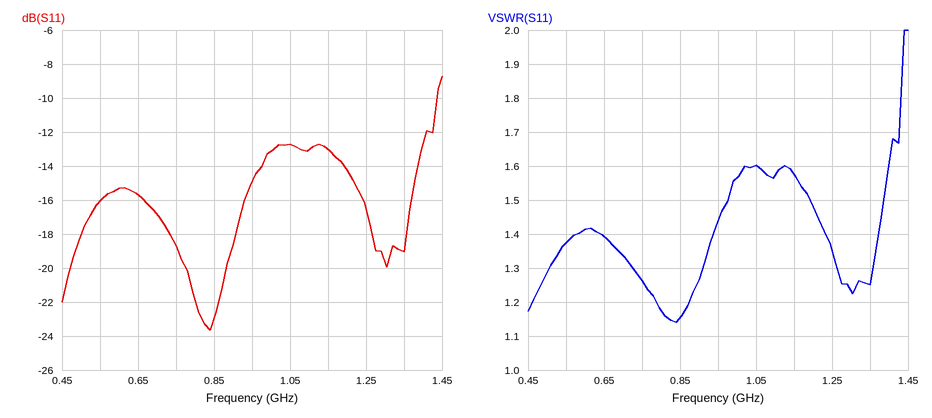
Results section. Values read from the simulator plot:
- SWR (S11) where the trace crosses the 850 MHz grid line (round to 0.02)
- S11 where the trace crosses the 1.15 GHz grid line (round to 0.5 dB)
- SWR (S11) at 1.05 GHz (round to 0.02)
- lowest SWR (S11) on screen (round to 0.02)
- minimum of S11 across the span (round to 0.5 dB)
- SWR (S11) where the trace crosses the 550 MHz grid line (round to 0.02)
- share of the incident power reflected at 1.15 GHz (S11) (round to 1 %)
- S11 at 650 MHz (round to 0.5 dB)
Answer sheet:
1.16
-13.0 dB
1.60
1.14
-23.5 dB
1.38
5 %
-15.5 dB
